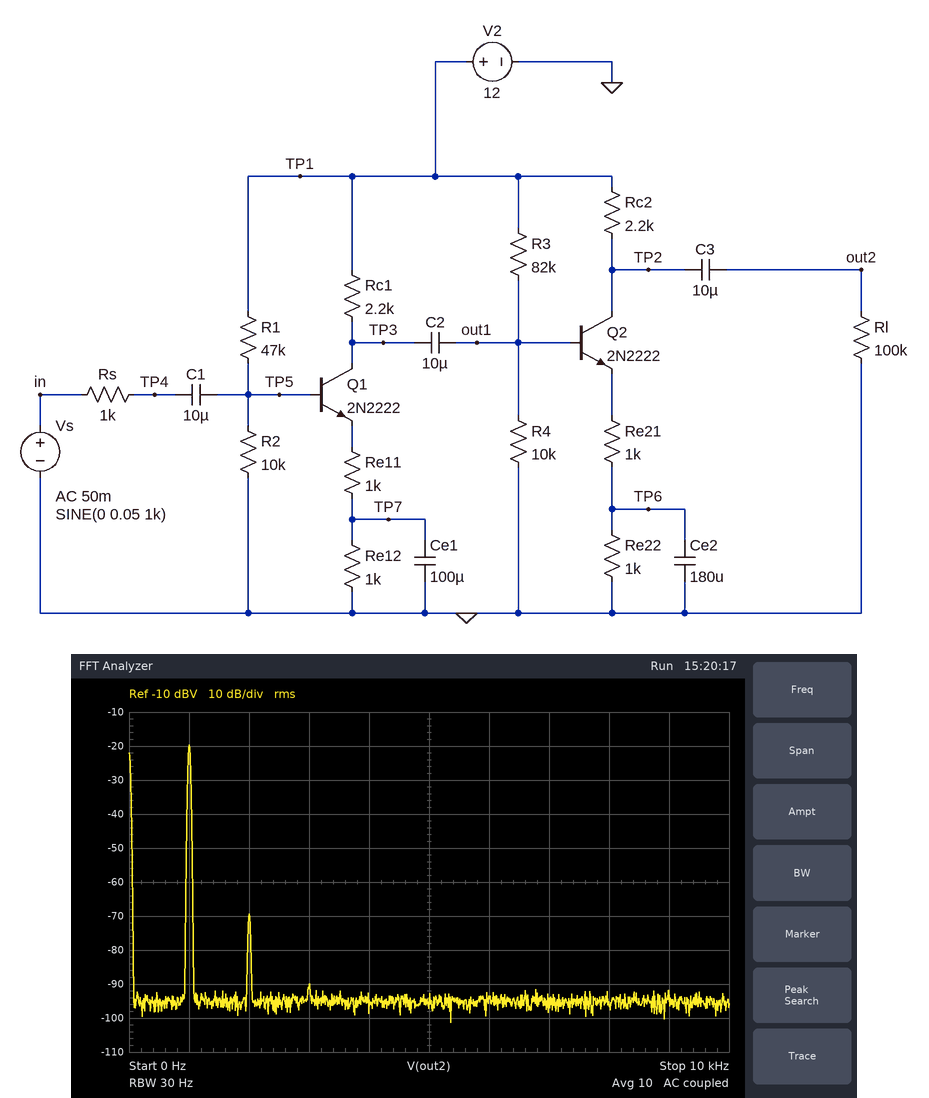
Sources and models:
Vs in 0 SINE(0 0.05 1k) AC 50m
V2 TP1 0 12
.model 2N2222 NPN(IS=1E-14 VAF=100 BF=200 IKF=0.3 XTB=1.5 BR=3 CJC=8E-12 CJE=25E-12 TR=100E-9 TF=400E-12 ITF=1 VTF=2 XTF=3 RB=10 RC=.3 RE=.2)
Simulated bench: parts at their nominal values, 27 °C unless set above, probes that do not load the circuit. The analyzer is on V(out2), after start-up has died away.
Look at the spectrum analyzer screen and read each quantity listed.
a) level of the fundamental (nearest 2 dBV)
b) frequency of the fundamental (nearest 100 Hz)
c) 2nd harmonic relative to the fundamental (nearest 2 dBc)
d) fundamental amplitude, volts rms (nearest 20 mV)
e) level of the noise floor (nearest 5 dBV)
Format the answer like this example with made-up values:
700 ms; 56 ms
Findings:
-20 dBV; 1.0 kHz; -50 dBc; 100 mV; -95 dBV
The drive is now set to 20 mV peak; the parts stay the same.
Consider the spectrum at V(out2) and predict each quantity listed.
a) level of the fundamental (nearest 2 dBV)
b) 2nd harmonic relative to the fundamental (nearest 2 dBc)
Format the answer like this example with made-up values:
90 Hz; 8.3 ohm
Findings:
-28 dBV; -58 dBc
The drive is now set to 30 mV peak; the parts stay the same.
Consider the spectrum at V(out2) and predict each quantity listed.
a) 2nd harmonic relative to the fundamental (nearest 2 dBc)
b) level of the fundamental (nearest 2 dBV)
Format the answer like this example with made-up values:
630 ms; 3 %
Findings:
-54 dBc; -24 dBV
